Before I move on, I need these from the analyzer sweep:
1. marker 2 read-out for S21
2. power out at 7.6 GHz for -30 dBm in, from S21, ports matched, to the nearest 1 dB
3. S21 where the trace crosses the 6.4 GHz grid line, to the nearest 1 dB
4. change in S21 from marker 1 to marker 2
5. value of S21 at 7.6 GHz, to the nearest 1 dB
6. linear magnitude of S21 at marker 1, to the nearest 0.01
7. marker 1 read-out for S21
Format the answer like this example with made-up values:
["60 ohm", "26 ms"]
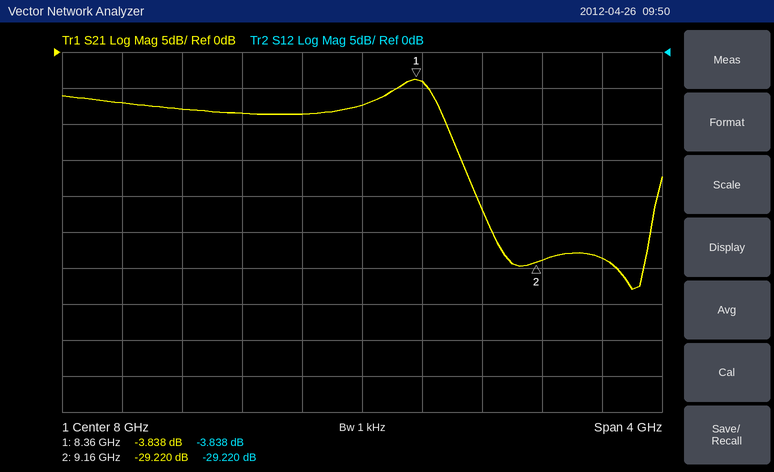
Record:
["-29.220 dB", "-39 dBm", "-7 dB", "-25.382 dB", "-9 dB", "0.64", "-3.838 dB"]
